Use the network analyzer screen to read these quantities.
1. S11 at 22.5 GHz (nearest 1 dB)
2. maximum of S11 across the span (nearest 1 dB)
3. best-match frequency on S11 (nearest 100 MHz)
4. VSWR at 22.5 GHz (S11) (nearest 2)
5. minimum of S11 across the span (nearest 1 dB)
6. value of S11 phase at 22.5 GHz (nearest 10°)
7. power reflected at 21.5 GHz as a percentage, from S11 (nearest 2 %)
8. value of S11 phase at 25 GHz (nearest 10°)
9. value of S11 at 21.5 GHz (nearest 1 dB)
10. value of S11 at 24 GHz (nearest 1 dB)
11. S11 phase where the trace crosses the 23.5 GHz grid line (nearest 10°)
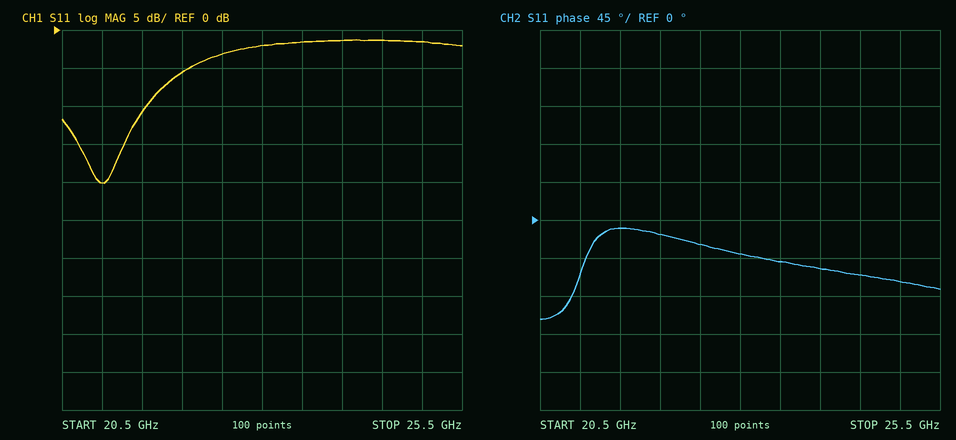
-3 dB
-1 dB
21.0 GHz
6
-20 dB
-30°
8 %
-70°
-11 dB
-1 dB
-50°
